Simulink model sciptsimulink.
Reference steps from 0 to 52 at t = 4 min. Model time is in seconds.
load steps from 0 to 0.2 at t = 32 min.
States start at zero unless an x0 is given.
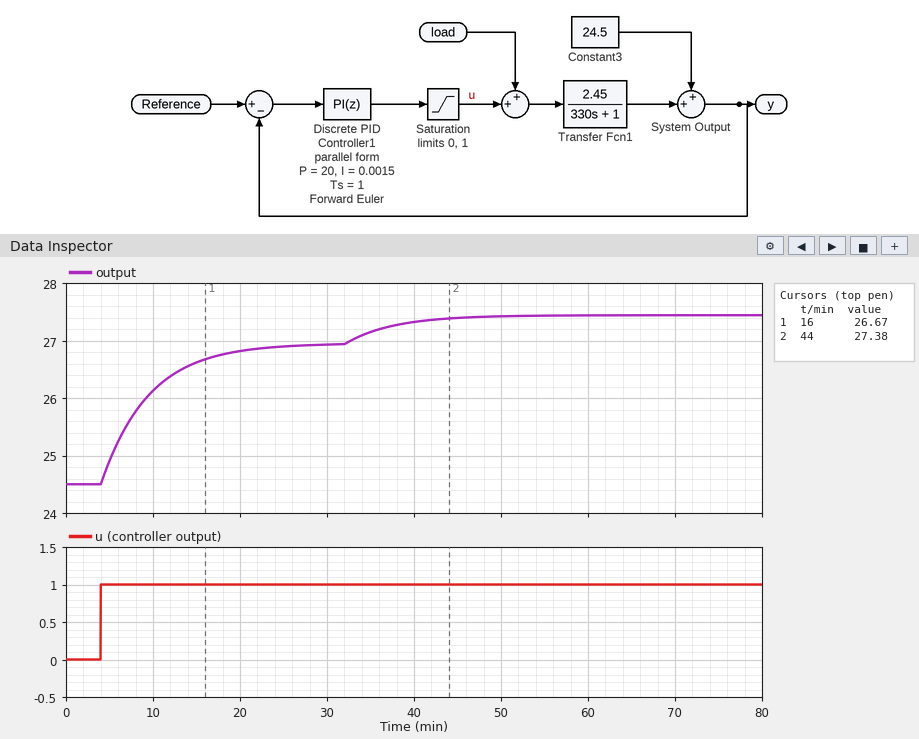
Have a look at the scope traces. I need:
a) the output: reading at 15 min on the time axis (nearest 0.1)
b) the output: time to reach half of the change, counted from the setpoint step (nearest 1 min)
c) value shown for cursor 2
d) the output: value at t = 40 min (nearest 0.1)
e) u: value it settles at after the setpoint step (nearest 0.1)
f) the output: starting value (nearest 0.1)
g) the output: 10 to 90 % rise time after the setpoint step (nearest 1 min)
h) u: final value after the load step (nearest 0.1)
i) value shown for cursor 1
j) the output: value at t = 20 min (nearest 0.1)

26.6
4 min
27.38
27.3
1.0
24.5
12 min
1.0
26.67
26.8
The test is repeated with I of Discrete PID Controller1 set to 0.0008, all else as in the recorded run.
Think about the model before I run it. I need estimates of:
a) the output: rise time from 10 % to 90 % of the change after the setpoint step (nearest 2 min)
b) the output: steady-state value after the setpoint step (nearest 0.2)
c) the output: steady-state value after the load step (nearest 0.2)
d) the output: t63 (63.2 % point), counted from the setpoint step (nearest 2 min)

12 min
27.0
27.4
6 min
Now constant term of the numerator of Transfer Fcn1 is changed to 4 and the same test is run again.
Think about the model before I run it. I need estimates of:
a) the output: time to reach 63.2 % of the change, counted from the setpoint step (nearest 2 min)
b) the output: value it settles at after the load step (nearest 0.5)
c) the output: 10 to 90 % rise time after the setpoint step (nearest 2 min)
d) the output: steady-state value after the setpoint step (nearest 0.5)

6 min
29.5
12 min
28.5
